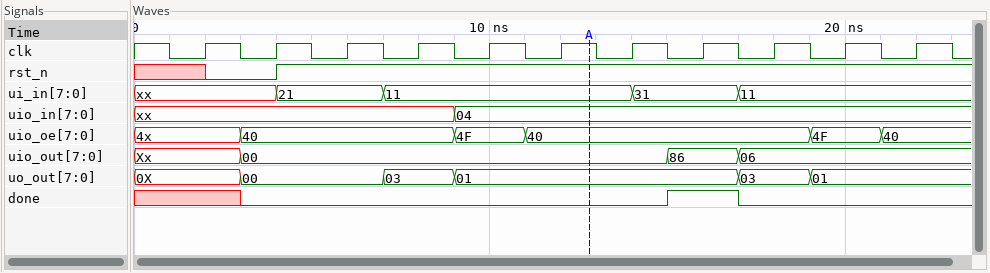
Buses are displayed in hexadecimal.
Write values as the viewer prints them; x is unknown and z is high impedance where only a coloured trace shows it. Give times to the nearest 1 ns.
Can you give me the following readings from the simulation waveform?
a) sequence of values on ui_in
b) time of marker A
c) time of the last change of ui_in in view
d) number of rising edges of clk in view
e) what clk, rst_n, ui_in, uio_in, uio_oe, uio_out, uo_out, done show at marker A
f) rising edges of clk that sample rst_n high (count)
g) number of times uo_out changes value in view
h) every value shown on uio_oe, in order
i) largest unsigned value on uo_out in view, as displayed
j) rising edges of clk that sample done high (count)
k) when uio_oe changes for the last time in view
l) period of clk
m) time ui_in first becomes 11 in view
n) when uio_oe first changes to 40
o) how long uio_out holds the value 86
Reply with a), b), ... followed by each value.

a) xx, 21, 11, 31, 11
b) 13 ns
c) 17 ns
d) 11
e) clk=1, rst_n=1, ui_in=11, uio_in=04, uio_oe=40, uio_out=00, uo_out=01, done=0
f) 9
g) 5
h) 4x, 40, 4F, 40, 4F, 40
i) 03
j) 1
k) 21 ns
l) 2 ns
m) 7 ns
n) 3 ns
o) 2 ns
